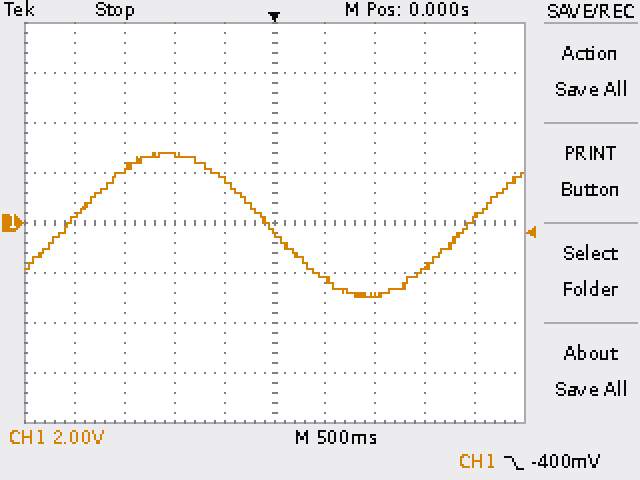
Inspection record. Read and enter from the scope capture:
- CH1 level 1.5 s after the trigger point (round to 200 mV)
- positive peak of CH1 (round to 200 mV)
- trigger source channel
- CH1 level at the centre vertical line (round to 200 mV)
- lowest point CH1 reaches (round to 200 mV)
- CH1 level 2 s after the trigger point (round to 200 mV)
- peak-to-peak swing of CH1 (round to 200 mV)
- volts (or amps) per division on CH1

-1.8 V
2.8 V
CH1
-400 mV
-3.0 V
200 mV
5.8 V
2 V
